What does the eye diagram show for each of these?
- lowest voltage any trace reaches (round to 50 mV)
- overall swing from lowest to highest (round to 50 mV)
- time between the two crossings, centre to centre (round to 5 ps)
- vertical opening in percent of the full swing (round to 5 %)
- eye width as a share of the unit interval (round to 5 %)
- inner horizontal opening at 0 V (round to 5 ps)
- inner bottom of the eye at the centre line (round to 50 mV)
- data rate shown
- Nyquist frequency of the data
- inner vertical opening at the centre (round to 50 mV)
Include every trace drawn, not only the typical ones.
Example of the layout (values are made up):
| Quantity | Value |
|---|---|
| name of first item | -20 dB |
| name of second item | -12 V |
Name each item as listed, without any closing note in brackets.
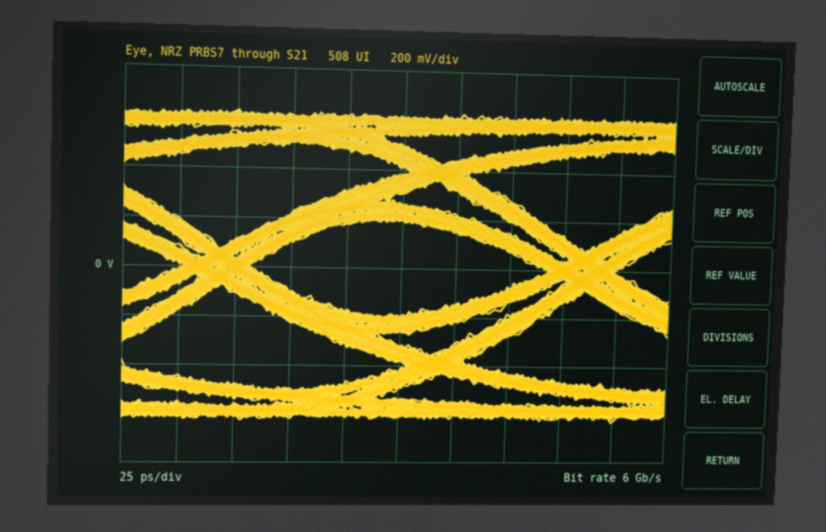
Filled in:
| Quantity | Value |
|---|---|
| lowest voltage any trace reaches | -650 mV |
| overall swing from lowest to highest | 1.25 V |
| time between the two crossings, centre to centre | 165 ps |
| vertical opening in percent of the full swing | 30 % |
| eye width as a share of the unit interval | 80 % |
| inner horizontal opening at 0 V | 135 ps |
| inner bottom of the eye at the centre line | -200 mV |
| data rate shown | 6 Gb/s |
| Nyquist frequency of the data | 3 GHz |
| inner vertical opening at the centre | 400 mV |
